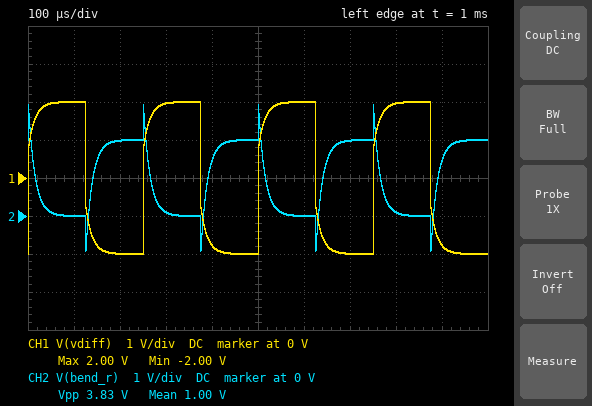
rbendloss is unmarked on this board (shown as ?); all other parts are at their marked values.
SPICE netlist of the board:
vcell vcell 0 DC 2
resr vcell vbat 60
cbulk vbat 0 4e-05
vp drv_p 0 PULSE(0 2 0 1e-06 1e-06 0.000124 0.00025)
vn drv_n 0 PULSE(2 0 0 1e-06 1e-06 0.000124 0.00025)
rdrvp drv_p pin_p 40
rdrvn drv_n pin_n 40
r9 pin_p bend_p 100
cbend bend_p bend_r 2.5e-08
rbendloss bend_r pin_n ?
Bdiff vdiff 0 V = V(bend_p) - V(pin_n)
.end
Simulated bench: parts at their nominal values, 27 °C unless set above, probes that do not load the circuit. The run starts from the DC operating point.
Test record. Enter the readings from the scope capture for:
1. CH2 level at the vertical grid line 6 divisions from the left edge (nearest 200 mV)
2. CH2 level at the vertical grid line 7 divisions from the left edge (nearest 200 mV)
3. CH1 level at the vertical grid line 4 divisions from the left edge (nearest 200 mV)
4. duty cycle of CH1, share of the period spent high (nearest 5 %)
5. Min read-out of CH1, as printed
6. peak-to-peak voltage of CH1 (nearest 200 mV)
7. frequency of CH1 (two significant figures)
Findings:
0 V
2.0 V
-1.8 V
50 %
-2.00 V
4.0 V
4.0 kHz
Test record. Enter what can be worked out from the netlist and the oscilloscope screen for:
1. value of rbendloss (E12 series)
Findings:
390 Ω
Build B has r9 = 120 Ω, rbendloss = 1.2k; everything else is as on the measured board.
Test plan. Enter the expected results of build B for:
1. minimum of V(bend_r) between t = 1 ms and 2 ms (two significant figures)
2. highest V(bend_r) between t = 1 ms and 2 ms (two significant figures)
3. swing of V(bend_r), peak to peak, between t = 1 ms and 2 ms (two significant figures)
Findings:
-1.4 V
3.4 V
4.8 V
